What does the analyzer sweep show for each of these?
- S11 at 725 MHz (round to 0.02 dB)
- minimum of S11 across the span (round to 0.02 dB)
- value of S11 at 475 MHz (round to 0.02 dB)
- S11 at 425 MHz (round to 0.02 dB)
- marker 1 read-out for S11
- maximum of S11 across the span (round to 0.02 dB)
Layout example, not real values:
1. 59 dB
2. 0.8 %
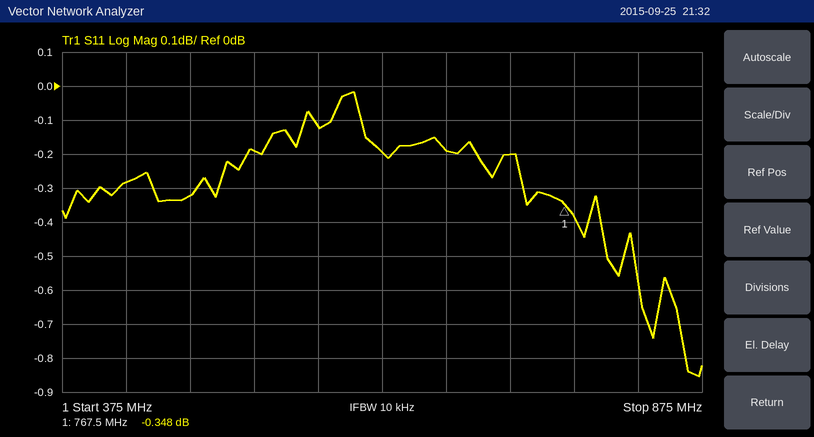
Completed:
1. -0.20 dB
2. -0.86 dB
3. -0.32 dB
4. -0.28 dB
5. -0.348 dB
6. -0.02 dB
